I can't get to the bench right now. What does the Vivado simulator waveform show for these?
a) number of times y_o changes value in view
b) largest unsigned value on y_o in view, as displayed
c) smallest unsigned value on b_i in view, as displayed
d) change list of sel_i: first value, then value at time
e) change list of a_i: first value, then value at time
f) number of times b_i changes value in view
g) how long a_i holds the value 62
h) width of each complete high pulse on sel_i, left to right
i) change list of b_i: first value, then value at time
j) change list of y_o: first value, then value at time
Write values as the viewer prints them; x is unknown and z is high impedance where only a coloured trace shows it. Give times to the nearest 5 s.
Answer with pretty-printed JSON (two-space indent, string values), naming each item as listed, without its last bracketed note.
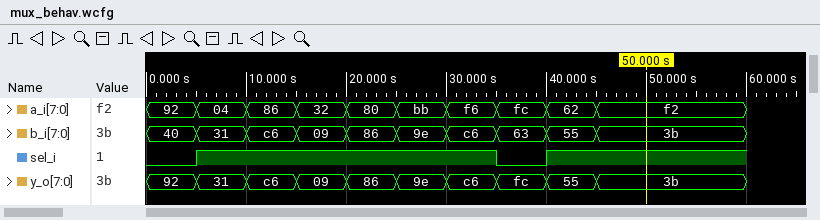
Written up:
{
  "number of times y_o changes value in view": "9",
  "largest unsigned value on y_o in view, as displayed": "fc",
  "smallest unsigned value on b_i in view, as displayed": "09",
  "change list of sel_i: first value, then value at time": "0, 1 at 5 s, 0 at 35 s, 1 at 40 s",
  "change list of a_i: first value, then value at time": "92, 04 at 5 s, 86 at 10 s, 32 at 15 s, 80 at 20 s, bb at 25 s, f6 at 30 s, fc at 35 s, 62 at 40 s, f2 at 45 s",
  "number of times b_i changes value in view": "9",
  "how long a_i holds the value 62": "5 s",
  "width of each complete high pulse on sel_i, left to right": "30 s",
  "change list of b_i: first value, then value at time": "40, 31 at 5 s, c6 at 10 s, 09 at 15 s, 86 at 20 s, 9e at 25 s, c6 at 30 s, 63 at 35 s, 55 at 40 s, 3b at 45 s",
  "change list of y_o: first value, then value at time": "92, 31 at 5 s, c6 at 10 s, 09 at 15 s, 86 at 20 s, 9e at 25 s, c6 at 30 s, fc at 35 s, 55 at 40 s, 3b at 45 s"
}
